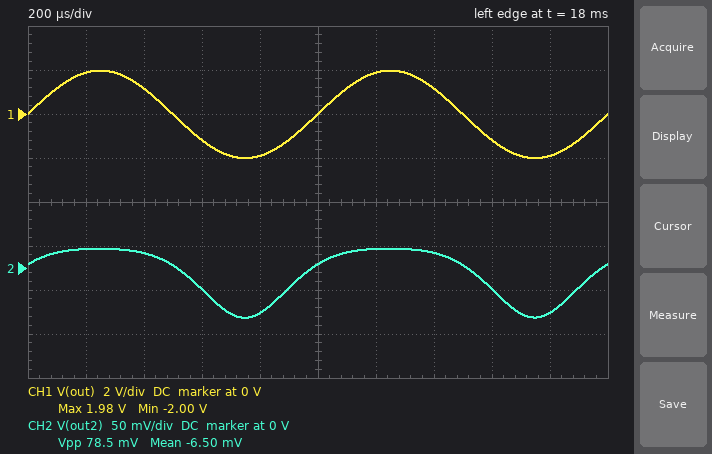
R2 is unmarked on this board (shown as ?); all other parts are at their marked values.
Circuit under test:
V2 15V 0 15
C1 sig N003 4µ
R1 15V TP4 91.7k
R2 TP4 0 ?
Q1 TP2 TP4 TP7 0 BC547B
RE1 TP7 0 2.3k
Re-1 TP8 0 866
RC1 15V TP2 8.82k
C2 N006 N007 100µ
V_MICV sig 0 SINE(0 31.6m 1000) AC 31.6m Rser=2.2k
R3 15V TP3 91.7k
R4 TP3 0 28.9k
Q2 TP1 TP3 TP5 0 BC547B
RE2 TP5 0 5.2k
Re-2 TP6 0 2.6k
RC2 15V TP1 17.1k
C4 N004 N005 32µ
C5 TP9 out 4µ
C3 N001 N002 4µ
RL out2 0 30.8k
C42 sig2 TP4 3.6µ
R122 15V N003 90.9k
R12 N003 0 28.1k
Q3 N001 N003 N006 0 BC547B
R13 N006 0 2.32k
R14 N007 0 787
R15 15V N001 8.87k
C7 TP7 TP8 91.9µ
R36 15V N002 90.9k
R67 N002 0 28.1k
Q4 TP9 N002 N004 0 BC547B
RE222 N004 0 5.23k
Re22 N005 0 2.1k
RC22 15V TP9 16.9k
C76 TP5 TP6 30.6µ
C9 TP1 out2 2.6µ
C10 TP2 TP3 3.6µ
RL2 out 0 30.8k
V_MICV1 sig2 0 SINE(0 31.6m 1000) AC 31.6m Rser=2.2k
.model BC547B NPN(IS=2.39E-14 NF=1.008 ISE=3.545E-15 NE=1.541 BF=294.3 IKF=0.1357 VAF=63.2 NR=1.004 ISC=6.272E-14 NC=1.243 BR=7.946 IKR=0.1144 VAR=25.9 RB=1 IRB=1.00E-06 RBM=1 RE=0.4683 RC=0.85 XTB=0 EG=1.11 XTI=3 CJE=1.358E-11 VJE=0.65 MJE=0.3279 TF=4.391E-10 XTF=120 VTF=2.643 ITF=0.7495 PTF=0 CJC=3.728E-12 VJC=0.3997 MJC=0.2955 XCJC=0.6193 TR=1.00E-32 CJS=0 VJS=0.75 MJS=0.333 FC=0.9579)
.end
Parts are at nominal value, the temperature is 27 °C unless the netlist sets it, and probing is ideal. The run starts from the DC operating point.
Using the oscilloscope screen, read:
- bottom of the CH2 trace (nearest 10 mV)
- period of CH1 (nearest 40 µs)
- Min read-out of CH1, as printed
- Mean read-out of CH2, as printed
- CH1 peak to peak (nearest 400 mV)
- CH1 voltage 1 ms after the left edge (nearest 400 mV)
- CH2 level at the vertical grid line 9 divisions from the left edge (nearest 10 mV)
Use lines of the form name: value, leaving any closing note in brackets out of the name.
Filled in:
bottom of the CH2 trace: -60 mV
period of CH1: 1.00 ms
Min read-out of CH1, as printed: -2.00 V
Mean read-out of CH2, as printed: -6.50 mV
CH1 peak to peak: 4.0 V
CH1 voltage 1 ms after the left edge: 0 V
CH2 level at the vertical grid line 9 divisions from the left edge: -50 mV
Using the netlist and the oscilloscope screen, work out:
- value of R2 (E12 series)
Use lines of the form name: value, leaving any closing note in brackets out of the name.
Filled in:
value of R2: 39 kΩ
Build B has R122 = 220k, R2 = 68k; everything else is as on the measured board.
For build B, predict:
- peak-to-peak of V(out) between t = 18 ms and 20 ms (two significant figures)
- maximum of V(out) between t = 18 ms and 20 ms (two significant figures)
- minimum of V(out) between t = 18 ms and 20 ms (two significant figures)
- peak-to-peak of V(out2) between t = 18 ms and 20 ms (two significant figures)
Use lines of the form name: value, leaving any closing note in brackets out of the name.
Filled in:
peak-to-peak of V(out) between t = 18 ms and 20 ms: 3.8 V
maximum of V(out) between t = 18 ms and 20 ms: 1.9 V
minimum of V(out) between t = 18 ms and 20 ms: -1.9 V
peak-to-peak of V(out2) between t = 18 ms and 20 ms: 34 mV
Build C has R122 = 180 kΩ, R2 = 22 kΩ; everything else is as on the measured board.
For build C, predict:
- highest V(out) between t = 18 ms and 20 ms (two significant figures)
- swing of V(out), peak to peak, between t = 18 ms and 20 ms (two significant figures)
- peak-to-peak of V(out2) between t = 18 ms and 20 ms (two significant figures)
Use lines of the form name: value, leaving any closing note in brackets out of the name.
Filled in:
highest V(out) between t = 18 ms and 20 ms: 1.9 V
swing of V(out), peak to peak, between t = 18 ms and 20 ms: 3.9 V
peak-to-peak of V(out2) between t = 18 ms and 20 ms: 3.2 V
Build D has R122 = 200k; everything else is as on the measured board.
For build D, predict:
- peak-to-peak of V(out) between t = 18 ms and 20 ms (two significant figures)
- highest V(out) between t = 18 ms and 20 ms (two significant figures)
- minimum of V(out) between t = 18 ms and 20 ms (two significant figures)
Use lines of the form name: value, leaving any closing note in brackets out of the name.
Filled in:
peak-to-peak of V(out) between t = 18 ms and 20 ms: 3.9 V
highest V(out) between t = 18 ms and 20 ms: 1.9 V
minimum of V(out) between t = 18 ms and 20 ms: -1.9 V
